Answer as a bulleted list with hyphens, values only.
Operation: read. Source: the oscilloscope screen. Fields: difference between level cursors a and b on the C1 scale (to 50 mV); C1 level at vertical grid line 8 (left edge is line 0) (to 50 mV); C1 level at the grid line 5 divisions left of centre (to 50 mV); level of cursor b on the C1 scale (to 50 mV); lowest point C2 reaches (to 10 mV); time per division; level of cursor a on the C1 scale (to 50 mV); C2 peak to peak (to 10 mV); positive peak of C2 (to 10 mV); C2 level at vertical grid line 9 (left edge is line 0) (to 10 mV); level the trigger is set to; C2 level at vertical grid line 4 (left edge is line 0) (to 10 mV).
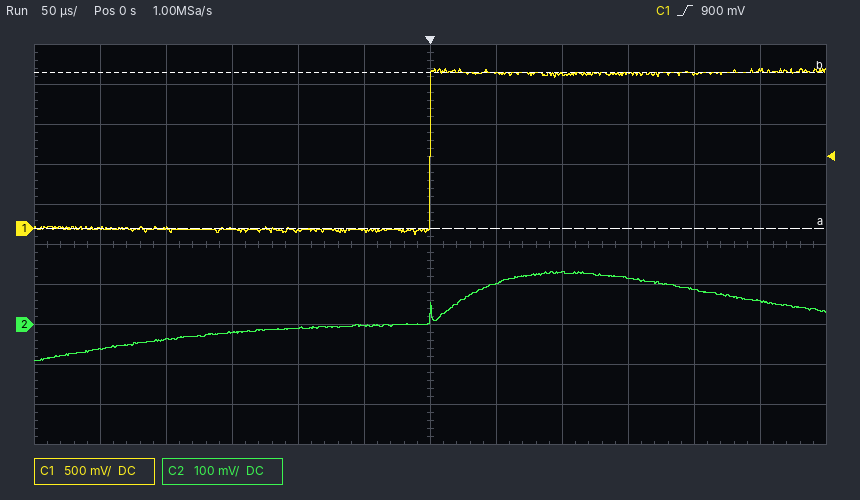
- 1.95 V
- 1.95 V
- 0 mV
- 1.95 V
- -90 mV
- 50 µs
- 0 mV
- 220 mV
- 130 mV
- 120 mV
- 900 mV
- -10 mV
